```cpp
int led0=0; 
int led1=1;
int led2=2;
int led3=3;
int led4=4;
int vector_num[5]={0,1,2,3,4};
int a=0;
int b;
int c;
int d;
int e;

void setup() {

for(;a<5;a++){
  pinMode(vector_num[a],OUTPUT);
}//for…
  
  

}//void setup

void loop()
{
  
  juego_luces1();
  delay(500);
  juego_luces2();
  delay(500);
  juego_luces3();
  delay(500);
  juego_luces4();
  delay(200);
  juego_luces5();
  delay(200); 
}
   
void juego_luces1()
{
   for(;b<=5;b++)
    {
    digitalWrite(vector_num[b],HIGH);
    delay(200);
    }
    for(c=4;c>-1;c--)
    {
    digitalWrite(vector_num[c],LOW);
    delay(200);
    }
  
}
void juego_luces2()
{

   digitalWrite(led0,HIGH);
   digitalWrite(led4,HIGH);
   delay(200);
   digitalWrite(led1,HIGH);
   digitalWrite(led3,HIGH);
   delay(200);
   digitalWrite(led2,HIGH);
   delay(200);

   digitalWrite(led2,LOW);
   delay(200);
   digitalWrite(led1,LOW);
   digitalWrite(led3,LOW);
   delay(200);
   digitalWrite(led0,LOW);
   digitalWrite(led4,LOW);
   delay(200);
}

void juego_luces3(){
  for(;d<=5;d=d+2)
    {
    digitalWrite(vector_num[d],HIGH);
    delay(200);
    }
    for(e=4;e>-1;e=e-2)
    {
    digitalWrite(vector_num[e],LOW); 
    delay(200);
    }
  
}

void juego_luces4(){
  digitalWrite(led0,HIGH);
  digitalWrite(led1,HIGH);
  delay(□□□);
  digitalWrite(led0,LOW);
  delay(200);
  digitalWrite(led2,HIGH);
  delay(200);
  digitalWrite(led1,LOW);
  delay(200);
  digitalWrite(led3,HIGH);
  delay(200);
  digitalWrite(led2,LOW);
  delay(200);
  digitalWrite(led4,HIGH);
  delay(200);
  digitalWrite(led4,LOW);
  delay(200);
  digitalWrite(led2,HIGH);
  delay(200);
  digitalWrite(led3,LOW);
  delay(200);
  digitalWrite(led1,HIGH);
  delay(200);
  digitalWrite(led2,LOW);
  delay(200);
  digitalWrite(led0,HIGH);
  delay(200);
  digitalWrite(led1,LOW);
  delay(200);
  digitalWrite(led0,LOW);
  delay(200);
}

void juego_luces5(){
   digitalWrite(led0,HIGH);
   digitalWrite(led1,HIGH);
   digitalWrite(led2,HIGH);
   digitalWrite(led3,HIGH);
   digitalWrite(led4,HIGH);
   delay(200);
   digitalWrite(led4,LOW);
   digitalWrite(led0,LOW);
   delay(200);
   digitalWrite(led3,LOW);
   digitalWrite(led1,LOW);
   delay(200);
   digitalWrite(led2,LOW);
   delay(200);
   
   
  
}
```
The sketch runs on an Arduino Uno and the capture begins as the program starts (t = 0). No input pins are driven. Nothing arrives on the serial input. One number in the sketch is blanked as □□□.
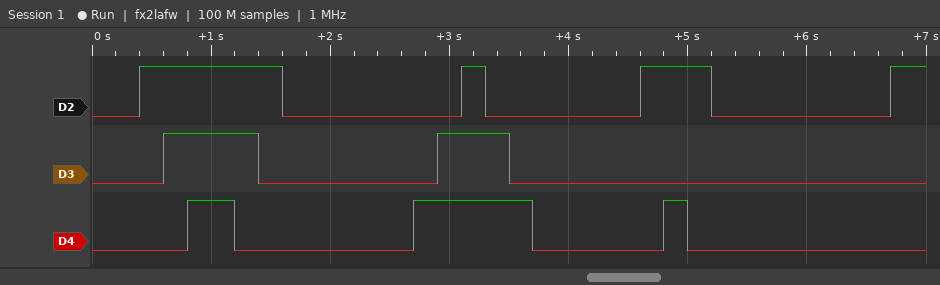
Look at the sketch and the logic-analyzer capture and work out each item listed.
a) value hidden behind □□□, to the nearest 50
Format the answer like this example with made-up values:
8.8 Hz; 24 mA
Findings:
400
